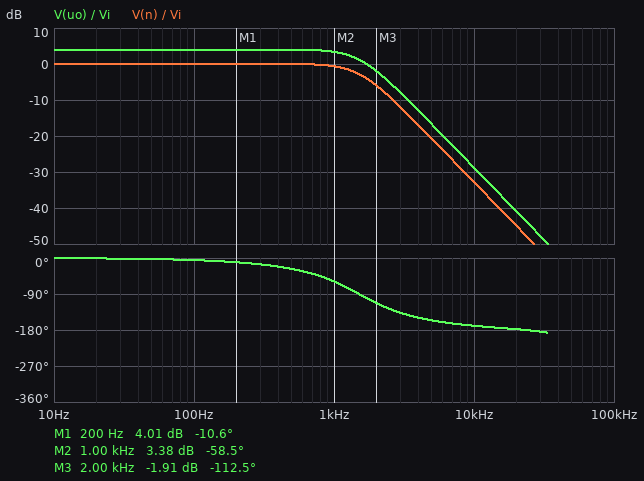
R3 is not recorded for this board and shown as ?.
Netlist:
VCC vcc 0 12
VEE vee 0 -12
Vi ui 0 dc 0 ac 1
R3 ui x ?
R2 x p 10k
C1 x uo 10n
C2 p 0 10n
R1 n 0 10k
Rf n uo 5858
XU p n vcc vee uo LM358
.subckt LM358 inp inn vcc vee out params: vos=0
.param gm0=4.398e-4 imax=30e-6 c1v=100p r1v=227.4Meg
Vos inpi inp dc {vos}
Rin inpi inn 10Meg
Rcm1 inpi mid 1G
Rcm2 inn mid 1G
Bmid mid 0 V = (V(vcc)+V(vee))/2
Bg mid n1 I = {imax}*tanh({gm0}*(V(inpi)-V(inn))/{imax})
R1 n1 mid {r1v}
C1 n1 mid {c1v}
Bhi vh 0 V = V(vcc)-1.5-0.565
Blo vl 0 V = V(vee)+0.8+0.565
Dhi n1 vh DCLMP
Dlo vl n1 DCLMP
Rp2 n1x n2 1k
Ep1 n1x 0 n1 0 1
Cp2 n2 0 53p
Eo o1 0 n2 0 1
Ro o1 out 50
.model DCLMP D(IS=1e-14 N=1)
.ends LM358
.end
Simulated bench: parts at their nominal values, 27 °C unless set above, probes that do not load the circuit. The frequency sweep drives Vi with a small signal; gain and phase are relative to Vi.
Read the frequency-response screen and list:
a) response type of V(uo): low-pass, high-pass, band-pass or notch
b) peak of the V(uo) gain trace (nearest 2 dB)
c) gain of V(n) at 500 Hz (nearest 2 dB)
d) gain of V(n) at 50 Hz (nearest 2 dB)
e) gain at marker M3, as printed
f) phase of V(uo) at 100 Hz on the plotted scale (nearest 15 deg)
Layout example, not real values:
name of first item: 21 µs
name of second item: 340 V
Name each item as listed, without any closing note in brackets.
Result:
response type of V(uo): low-pass, high-pass, band-pass or notch: low-pass
peak of the V(uo) gain trace: 4 dB
gain of V(n) at 500 Hz: 0 dB
gain of V(n) at 50 Hz: 0 dB
gain at marker M3, as printed: -1.91 dB
phase of V(uo) at 100 Hz on the plotted scale: 0 deg
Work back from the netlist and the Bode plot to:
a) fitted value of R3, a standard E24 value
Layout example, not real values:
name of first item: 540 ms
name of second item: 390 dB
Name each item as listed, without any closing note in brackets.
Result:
fitted value of R3, a standard E24 value: 11 kΩ
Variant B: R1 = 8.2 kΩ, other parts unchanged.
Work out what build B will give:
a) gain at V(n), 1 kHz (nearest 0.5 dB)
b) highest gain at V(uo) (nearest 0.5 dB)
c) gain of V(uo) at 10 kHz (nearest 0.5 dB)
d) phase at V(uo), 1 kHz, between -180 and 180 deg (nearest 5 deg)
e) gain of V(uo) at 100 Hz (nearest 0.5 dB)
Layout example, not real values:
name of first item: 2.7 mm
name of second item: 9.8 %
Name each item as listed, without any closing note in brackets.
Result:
gain at V(n), 1 kHz: 0 dB
highest gain at V(uo): 5.0 dB
gain of V(uo) at 10 kHz: -28.0 dB
phase at V(uo), 1 kHz, between -180 and 180 deg: -55 deg
gain of V(uo) at 100 Hz: 4.5 dB
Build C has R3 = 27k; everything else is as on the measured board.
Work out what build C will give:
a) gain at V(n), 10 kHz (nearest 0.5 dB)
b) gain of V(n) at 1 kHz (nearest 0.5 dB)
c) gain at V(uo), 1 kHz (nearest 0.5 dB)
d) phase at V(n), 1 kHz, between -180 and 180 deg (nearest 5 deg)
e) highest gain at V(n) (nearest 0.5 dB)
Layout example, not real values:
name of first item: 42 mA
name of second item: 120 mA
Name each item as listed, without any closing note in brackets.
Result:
gain at V(n), 10 kHz: -40.5 dB
gain of V(n) at 1 kHz: -2.5 dB
gain at V(uo), 1 kHz: 1.5 dB
phase at V(n), 1 kHz, between -180 and 180 deg: -95 deg
highest gain at V(n): 0 dB
